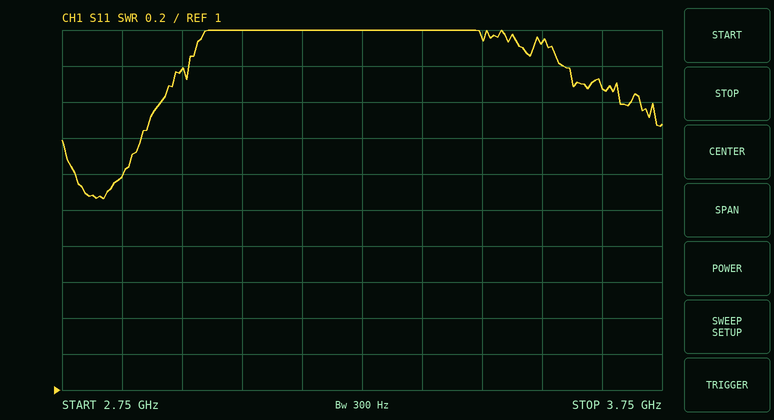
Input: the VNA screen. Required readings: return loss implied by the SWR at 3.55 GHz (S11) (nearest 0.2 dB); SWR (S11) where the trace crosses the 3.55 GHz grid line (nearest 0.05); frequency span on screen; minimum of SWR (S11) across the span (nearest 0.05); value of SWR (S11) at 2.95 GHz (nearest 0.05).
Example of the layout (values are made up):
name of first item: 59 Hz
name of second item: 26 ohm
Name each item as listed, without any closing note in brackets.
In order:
return loss implied by the SWR at 3.55 GHz (S11): 6.2 dB
SWR (S11) where the trace crosses the 3.55 GHz grid line: 2.95
frequency span on screen: 1 GHz
minimum of SWR (S11) across the span: 2.05
value of SWR (S11) at 2.95 GHz: 2.80
